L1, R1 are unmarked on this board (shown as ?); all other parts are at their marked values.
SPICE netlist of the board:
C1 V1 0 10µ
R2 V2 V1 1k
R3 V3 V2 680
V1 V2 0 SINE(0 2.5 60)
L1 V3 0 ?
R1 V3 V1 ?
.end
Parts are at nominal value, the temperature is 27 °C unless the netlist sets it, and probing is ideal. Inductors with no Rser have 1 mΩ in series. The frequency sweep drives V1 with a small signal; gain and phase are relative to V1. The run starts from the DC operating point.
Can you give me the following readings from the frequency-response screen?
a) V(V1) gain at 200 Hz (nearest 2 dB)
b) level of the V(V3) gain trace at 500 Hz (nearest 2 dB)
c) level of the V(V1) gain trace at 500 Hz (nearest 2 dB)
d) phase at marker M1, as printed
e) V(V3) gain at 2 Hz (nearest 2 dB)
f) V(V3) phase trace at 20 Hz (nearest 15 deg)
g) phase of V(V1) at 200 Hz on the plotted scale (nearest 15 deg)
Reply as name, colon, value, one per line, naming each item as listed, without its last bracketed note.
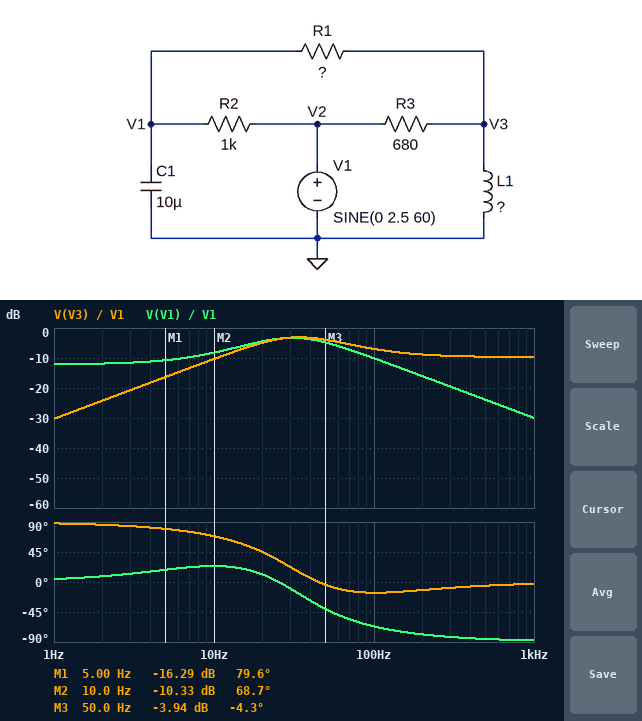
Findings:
V(V1) gain at 200 Hz: -16 dB
level of the V(V3) gain trace at 500 Hz: -10 dB
level of the V(V1) gain trace at 500 Hz: -24 dB
phase at marker M1, as printed: 79.6 deg
V(V3) gain at 2 Hz: -24 dB
V(V3) phase trace at 20 Hz: 45 deg
phase of V(V1) at 200 Hz on the plotted scale: -75 deg
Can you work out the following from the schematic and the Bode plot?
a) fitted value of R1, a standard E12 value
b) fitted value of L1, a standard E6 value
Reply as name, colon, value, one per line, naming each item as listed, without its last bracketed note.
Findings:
fitted value of R1, a standard E12 value: 330 Ω
fitted value of L1, a standard E6 value: 2.2 H
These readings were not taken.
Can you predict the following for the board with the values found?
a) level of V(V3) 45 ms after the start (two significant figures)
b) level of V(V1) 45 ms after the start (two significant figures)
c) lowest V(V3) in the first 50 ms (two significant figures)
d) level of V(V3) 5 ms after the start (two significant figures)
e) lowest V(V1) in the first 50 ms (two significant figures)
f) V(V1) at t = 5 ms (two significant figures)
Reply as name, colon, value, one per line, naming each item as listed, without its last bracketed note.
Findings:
level of V(V3) 45 ms after the start: -1.3 V
level of V(V1) 45 ms after the start: -470 mV
lowest V(V3) in the first 50 ms: -1.7 V
level of V(V3) 5 ms after the start: 1.1 V
lowest V(V1) in the first 50 ms: -1.4 V
V(V1) at t = 5 ms: 1.1 V
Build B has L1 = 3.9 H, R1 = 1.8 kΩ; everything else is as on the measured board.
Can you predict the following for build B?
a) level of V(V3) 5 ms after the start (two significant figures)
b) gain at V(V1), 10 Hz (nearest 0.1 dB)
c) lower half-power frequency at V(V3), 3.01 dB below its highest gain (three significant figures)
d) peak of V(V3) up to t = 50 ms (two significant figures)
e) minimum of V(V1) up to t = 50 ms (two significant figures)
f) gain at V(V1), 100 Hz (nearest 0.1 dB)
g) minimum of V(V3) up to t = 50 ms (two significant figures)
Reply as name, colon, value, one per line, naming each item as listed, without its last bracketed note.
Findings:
level of V(V3) 5 ms after the start: 1.3 V
gain at V(V1), 10 Hz: -3.5 dB
lower half-power frequency at V(V3), 3.01 dB below its highest gain: 14.1 Hz
peak of V(V3) up to t = 50 ms: 1.8 V
minimum of V(V1) up to t = 50 ms: -870 mV
gain at V(V1), 100 Hz: -13.3 dB
minimum of V(V3) up to t = 50 ms: -2.0 V
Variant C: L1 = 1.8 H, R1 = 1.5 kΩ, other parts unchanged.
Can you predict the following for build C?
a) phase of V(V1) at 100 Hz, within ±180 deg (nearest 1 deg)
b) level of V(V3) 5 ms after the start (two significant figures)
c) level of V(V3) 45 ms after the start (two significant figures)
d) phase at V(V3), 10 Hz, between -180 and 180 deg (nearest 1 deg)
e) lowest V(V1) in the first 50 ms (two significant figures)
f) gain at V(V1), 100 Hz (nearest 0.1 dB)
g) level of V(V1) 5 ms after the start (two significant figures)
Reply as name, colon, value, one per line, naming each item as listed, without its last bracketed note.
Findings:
phase of V(V1) at 100 Hz, within ±180 deg: -70 deg
level of V(V3) 5 ms after the start: 800 mV
level of V(V3) 45 ms after the start: -1.5 V
phase at V(V3), 10 Hz, between -180 and 180 deg: 74 deg
lowest V(V1) in the first 50 ms: -840 mV
gain at V(V1), 100 Hz: -13.2 dB
level of V(V1) 5 ms after the start: 850 mV
